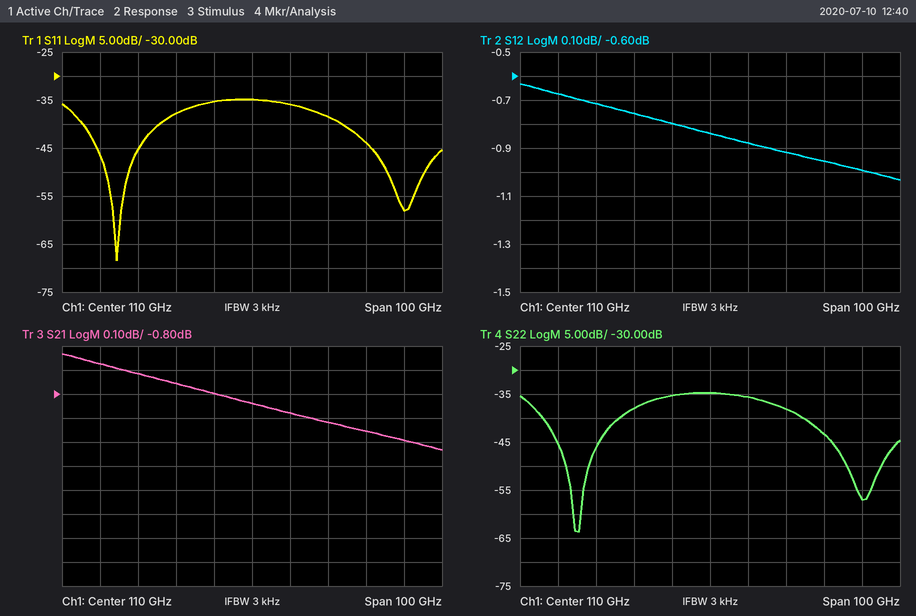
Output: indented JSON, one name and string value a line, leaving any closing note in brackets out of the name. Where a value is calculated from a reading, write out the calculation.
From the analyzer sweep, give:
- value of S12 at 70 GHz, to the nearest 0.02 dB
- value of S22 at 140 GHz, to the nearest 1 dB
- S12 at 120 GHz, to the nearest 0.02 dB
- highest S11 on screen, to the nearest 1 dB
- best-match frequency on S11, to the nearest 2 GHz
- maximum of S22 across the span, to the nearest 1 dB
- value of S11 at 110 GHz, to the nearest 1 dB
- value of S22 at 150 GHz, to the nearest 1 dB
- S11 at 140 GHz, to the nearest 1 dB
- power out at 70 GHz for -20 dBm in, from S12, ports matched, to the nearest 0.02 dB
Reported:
{
  "value of S12 at 70 GHz, to the nearest 0.02 dB": "-0.68 dB",
  "value of S22 at 140 GHz, to the nearest 1 dB": "-43 dB",
  "S12 at 120 GHz, to the nearest 0.02 dB": "-0.88 dB",
  "highest S11 on screen, to the nearest 1 dB": "-35 dB",
  "best-match frequency on S11, to the nearest 2 GHz": "74 GHz",
  "maximum of S22 across the span, to the nearest 1 dB": "-35 dB",
  "value of S11 at 110 GHz, to the nearest 1 dB": "-35 dB",
  "value of S22 at 150 GHz, to the nearest 1 dB": "-57 dB",
  "S11 at 140 GHz, to the nearest 1 dB": "-44 dB",
  "power out at 70 GHz for -20 dBm in, from S12, ports matched, to the nearest 0.02 dB": "-20 dBm + (-0.68 dB) = -20.68 dBm"
}
